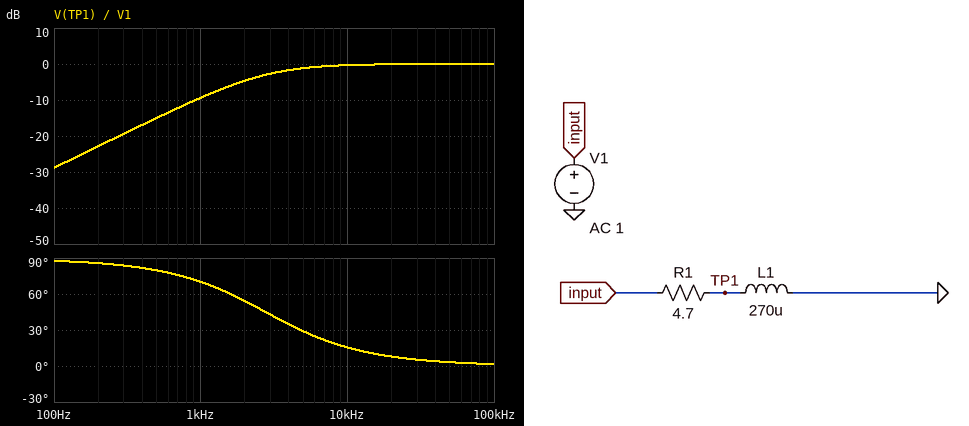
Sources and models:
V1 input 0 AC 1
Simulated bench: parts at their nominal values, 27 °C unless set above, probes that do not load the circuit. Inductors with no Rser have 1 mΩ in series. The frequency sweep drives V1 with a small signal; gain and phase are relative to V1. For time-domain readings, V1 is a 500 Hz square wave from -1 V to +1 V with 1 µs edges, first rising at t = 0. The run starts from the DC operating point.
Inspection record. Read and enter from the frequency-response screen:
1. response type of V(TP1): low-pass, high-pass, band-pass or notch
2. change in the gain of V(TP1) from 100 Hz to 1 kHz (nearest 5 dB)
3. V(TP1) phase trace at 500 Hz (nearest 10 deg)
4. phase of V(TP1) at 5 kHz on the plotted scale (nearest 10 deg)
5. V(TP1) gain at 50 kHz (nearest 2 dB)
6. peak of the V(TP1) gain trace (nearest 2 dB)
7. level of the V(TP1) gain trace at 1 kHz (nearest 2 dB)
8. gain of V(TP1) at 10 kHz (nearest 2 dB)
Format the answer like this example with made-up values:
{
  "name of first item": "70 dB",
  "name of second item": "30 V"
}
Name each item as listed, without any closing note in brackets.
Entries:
{
  "response type of V(TP1): low-pass, high-pass, band-pass or notch": "high-pass",
  "change in the gain of V(TP1) from 100 Hz to 1 kHz": "20 dB",
  "V(TP1) phase trace at 500 Hz": "80 deg",
  "phase of V(TP1) at 5 kHz on the plotted scale": "30 deg",
  "V(TP1) gain at 50 kHz": "0 dB",
  "peak of the V(TP1) gain trace": "0 dB",
  "level of the V(TP1) gain trace at 1 kHz": "-10 dB",
  "gain of V(TP1) at 10 kHz": "0 dB"
}
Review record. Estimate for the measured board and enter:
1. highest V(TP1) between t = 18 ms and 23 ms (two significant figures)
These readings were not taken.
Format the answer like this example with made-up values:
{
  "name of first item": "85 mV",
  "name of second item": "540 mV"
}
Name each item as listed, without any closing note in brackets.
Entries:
{
  "highest V(TP1) between t = 18 ms and 23 ms": "2.0 V"
}
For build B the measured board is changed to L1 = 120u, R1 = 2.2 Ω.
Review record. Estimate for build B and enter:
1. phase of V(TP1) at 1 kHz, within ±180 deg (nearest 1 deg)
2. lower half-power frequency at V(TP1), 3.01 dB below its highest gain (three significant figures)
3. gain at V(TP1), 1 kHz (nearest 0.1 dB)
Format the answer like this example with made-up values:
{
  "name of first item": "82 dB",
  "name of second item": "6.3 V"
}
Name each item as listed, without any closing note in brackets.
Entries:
{
  "phase of V(TP1) at 1 kHz, within ±180 deg": "71 deg",
  "lower half-power frequency at V(TP1), 3.01 dB below its highest gain": "2.92 kHz",
  "gain at V(TP1), 1 kHz": "-9.8 dB"
}
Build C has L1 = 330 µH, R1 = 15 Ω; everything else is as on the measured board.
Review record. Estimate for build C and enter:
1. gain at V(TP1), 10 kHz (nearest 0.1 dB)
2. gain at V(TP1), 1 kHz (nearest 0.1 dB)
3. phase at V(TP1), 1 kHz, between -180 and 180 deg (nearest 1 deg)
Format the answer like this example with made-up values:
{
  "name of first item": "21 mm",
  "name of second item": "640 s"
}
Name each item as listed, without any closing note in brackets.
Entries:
{
  "gain at V(TP1), 10 kHz": "-1.8 dB",
  "gain at V(TP1), 1 kHz": "-17.3 dB",
  "phase at V(TP1), 1 kHz, between -180 and 180 deg": "82 deg"
}
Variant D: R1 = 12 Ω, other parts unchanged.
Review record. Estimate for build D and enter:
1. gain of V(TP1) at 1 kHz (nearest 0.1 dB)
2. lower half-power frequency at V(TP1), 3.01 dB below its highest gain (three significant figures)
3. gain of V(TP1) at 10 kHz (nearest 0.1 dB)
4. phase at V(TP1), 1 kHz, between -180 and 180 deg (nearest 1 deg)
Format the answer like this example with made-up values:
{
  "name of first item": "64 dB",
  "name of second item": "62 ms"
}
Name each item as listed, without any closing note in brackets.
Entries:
{
  "gain of V(TP1) at 1 kHz": "-17.1 dB",
  "lower half-power frequency at V(TP1), 3.01 dB below its highest gain": "7.07 kHz",
  "gain of V(TP1) at 10 kHz": "-1.8 dB",
  "phase at V(TP1), 1 kHz, between -180 and 180 deg": "82 deg"
}
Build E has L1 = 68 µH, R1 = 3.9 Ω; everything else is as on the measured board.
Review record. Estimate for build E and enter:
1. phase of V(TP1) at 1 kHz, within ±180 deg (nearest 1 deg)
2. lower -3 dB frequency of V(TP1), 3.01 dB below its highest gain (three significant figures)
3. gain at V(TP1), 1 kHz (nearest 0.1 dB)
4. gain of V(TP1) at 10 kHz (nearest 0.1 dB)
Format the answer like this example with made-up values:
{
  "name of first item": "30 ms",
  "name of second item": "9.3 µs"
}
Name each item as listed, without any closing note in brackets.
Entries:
{
  "phase of V(TP1) at 1 kHz, within ±180 deg": "84 deg",
  "lower -3 dB frequency of V(TP1), 3.01 dB below its highest gain": "9.13 kHz",
  "gain at V(TP1), 1 kHz": "-19.3 dB",
  "gain of V(TP1) at 10 kHz": "-2.6 dB"
}
